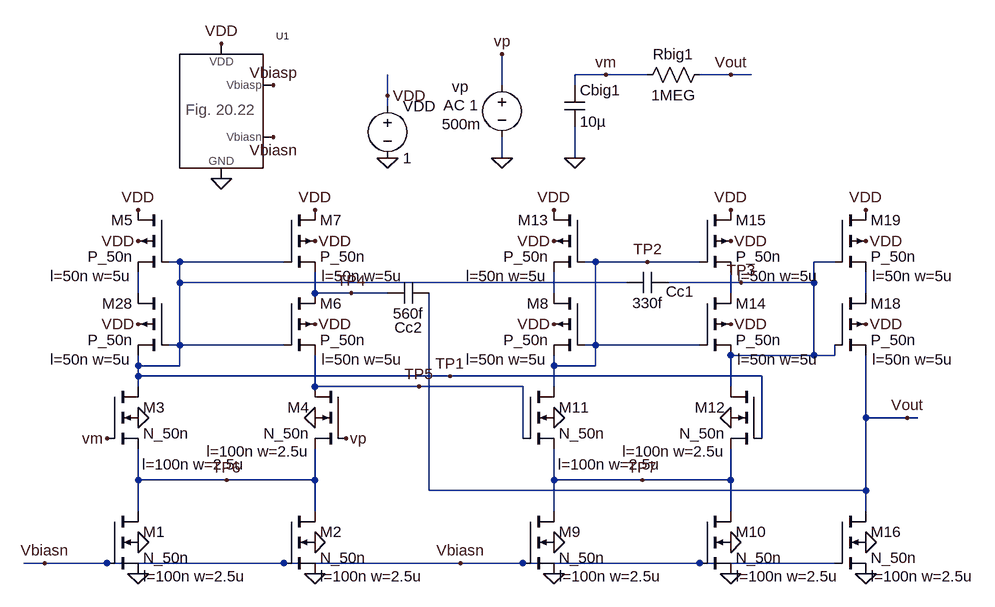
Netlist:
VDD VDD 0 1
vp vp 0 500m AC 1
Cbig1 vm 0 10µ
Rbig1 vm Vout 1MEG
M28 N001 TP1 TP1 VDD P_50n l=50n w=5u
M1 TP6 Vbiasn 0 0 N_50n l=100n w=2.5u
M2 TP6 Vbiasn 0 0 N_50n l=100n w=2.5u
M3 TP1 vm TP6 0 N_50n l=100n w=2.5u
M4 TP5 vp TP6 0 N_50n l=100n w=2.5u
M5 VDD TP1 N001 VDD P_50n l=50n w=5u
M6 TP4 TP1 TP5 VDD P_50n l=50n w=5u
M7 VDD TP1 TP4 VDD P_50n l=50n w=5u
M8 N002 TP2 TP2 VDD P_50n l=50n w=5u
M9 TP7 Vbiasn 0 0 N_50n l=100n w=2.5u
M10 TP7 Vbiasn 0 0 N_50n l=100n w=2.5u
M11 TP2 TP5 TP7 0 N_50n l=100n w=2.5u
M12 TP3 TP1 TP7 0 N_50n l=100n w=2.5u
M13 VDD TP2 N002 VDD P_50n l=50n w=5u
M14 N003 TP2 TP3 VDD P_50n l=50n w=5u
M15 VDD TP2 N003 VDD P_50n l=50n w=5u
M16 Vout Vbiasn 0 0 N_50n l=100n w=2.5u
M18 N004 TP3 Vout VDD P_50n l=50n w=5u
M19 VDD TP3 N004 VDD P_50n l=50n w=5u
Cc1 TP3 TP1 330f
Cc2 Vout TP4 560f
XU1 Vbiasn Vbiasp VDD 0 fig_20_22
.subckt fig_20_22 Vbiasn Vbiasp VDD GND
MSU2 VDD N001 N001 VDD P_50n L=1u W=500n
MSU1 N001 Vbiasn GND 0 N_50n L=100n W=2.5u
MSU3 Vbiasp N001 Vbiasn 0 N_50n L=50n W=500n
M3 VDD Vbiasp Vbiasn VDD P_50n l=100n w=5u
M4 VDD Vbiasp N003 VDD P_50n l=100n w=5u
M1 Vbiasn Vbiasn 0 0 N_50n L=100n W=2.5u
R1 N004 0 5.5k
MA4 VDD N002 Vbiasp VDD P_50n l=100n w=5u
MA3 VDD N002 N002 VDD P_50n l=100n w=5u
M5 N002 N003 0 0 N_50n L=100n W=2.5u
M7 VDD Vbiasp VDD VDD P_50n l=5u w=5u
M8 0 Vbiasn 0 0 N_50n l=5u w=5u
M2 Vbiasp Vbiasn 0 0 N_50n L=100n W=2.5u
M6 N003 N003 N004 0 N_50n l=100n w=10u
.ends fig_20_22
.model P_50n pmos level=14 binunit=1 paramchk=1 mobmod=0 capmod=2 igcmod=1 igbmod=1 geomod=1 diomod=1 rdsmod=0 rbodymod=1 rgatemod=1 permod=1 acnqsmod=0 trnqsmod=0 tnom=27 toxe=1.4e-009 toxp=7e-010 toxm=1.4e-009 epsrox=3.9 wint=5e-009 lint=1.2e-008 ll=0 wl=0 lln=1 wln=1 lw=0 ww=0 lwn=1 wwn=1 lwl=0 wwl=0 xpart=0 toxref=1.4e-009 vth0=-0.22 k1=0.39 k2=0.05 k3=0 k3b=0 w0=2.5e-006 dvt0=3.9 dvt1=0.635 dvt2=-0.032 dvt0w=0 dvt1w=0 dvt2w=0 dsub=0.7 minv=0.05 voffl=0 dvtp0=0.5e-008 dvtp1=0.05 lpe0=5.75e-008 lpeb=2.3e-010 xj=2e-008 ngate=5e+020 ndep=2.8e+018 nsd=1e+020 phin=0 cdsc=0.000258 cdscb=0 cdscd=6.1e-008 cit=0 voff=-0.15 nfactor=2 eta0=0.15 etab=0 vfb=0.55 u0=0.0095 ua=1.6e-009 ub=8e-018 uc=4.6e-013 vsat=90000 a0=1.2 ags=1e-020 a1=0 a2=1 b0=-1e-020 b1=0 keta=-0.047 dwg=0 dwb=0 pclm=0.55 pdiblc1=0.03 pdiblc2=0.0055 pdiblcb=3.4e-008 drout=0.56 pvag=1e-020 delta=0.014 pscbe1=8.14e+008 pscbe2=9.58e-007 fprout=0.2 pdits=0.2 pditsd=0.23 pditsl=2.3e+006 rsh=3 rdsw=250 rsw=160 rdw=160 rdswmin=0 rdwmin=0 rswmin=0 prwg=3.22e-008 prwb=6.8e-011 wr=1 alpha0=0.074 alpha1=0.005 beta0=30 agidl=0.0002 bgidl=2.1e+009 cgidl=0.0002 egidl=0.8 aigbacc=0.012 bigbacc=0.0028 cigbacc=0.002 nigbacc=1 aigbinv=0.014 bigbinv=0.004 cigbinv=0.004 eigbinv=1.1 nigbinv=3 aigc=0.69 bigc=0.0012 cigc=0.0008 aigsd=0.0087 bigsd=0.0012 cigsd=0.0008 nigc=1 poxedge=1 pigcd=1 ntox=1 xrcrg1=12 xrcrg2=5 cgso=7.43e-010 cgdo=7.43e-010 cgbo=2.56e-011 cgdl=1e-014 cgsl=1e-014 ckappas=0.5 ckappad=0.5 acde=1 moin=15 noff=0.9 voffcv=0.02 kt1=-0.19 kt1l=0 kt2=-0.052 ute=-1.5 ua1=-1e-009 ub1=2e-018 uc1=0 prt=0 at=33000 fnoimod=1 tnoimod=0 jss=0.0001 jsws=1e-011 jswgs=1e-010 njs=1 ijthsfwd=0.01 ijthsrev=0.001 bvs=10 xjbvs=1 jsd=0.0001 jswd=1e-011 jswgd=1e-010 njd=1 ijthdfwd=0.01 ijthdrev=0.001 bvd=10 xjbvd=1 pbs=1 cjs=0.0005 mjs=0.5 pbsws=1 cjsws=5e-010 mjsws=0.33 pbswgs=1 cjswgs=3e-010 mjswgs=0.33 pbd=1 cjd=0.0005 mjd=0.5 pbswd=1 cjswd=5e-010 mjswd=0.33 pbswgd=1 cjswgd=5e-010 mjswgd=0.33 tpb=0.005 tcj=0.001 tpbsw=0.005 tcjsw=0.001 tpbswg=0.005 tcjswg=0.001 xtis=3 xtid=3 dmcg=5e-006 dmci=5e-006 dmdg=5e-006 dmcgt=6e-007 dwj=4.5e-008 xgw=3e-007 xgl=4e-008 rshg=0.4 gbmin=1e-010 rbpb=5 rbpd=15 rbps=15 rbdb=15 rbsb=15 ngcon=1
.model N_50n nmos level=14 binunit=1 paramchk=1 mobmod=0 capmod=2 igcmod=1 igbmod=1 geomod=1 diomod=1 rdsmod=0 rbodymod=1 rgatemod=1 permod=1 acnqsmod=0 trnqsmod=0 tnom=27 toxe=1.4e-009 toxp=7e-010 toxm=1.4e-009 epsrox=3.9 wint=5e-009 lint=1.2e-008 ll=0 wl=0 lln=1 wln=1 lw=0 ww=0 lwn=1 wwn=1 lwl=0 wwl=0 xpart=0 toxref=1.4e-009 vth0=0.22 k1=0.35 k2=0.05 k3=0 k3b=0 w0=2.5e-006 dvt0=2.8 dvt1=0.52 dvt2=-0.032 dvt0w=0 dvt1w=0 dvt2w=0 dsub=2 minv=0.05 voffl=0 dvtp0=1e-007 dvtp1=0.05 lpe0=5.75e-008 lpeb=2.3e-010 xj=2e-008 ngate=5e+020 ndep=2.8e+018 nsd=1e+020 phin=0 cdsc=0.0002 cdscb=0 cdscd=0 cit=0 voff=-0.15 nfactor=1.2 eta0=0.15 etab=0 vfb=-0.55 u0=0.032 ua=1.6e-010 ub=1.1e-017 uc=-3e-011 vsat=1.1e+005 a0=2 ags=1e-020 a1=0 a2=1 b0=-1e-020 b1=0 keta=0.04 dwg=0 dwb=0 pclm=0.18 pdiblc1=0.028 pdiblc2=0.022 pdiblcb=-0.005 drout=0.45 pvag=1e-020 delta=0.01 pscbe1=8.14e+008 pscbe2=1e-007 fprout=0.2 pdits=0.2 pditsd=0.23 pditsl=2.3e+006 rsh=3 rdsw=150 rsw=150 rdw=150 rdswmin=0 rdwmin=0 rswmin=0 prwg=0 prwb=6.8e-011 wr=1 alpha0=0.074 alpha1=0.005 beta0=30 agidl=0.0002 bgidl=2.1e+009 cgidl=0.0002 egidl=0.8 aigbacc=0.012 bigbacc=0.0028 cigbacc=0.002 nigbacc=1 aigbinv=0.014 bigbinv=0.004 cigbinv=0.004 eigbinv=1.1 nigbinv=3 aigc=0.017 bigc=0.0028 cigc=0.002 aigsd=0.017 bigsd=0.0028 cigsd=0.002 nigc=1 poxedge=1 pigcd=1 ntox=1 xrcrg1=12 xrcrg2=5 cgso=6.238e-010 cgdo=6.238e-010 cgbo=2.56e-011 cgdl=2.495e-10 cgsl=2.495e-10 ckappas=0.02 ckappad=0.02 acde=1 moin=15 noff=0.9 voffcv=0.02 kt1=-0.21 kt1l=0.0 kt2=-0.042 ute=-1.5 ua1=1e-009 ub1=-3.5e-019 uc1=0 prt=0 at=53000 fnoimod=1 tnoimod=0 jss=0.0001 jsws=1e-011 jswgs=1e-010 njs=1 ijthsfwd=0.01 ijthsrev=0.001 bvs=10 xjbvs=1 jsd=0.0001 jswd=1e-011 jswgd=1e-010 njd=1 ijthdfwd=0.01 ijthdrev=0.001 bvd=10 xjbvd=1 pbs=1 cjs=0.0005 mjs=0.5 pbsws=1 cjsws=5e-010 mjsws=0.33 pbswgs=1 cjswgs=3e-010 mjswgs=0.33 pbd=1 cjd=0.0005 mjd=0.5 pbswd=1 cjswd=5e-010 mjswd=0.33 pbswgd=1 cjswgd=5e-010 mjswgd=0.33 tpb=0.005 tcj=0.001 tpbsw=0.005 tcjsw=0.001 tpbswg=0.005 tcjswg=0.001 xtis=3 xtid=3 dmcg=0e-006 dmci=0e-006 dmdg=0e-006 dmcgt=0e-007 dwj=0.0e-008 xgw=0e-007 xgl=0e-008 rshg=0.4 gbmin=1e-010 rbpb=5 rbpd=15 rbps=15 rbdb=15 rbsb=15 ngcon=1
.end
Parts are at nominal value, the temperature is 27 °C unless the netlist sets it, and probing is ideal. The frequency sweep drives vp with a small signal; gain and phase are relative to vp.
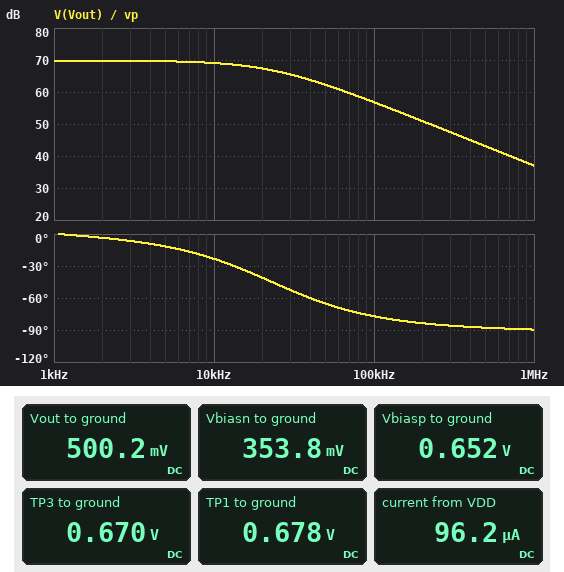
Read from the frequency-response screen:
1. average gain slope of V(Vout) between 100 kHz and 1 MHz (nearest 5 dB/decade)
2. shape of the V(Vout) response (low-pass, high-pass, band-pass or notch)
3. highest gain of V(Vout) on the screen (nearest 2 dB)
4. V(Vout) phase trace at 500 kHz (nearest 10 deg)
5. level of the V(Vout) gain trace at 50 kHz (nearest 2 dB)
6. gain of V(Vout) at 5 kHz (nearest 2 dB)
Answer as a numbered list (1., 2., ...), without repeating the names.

1. -20 dB/decade
2. low-pass
3. 70 dB
4. -90 deg
5. 62 dB
6. 70 dB
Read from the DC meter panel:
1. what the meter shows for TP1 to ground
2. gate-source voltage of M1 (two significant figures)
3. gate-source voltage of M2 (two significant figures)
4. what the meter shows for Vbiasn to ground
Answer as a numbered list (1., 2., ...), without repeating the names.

1. 0.678 V
2. 350 mV
3. 350 mV
4. 353.8 mV
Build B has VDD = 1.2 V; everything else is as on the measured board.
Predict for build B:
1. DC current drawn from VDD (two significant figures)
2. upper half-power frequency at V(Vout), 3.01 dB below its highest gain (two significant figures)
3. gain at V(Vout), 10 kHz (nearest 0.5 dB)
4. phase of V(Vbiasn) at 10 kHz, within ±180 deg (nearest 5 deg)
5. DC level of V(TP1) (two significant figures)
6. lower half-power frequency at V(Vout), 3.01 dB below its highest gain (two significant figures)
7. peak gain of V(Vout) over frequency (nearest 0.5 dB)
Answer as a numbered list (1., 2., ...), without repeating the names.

1. 100 µA
2. 21 kHz
3. 70.0 dB
4. 25 deg
5. 880 mV
6. 55 Hz
7. 71.0 dB
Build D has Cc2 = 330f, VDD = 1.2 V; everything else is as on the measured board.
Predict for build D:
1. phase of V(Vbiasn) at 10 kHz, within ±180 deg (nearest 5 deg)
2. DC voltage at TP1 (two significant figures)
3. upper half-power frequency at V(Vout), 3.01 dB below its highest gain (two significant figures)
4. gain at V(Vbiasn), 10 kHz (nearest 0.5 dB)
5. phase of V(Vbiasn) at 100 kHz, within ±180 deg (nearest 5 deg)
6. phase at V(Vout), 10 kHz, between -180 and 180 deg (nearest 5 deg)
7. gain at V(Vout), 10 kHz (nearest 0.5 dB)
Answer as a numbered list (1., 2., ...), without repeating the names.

1. 35 deg
2. 880 mV
3. 34 kHz
4. -44.5 dB
5. 15 deg
6. -15 deg
7. 70.5 dB
